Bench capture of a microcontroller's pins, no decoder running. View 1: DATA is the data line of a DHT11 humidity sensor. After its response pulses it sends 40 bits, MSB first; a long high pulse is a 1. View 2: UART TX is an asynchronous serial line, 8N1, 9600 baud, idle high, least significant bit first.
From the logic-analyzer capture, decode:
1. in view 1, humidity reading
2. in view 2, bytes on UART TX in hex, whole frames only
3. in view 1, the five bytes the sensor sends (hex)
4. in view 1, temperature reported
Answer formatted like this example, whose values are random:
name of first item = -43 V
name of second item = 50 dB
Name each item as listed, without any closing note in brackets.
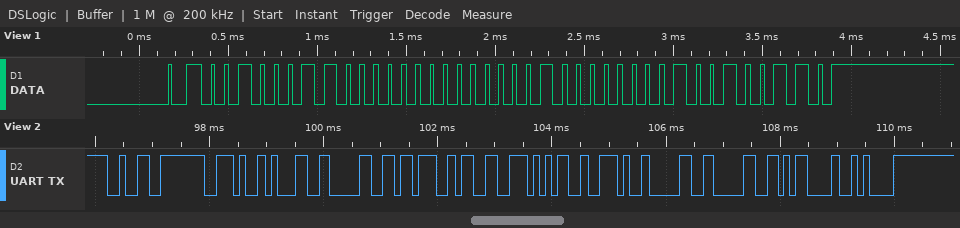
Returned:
in view 1, humidity reading = 35 %
in view 2, bytes on UART TX in hex, whole frames only = 0x32 0x2E 0x31 0x30 0x3B 0x33 0x35 0x2E 0x30 0x30 0x0D 0x0A
in view 1, the five bytes the sensor sends = 23 00 02 01 26
in view 1, temperature reported = 2.1 °C
